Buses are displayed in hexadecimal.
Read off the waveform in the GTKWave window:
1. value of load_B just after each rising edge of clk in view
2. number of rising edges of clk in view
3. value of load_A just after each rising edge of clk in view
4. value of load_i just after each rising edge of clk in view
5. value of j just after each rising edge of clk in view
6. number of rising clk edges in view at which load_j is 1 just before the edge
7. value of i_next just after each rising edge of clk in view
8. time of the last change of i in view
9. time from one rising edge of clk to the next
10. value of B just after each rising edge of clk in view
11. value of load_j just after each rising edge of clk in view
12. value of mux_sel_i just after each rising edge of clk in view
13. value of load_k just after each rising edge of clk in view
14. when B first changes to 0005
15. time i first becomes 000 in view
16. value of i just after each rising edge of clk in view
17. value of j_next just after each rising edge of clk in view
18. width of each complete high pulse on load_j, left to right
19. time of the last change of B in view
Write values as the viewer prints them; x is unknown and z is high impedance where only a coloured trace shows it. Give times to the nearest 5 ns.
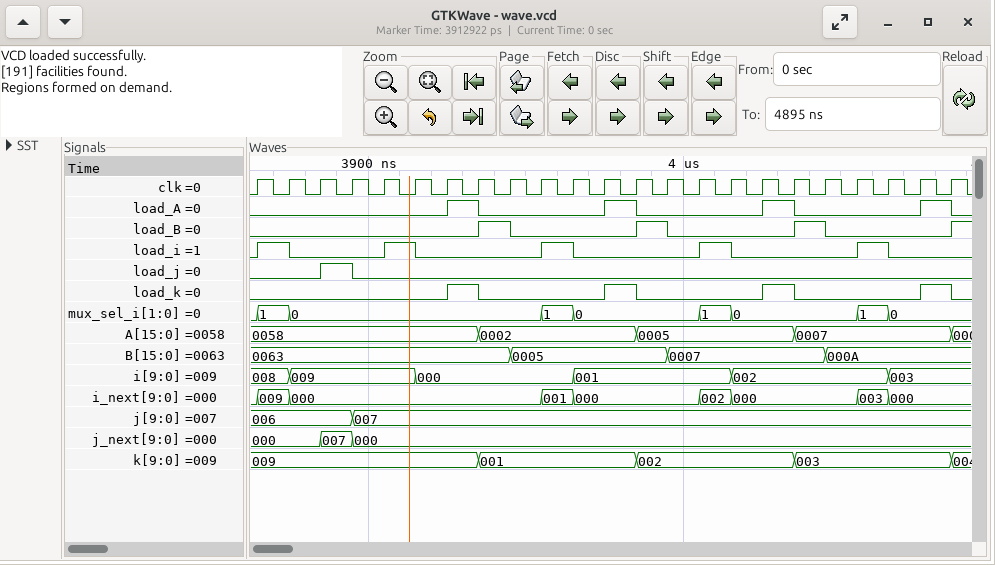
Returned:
0 0 0 0 0 0 0 1 0 0 0 0 1 0 0 0 0 1 0 0 0 0 1
23
0 0 0 0 0 0 1 0 0 0 0 1 0 0 0 0 1 0 0 0 0 1 0
1 0 0 0 1 0 0 0 0 1 0 0 0 0 1 0 0 0 0 1 0 0 0
006, 006, 006, 007, 007, 007, 007, 007, 007, 007, 007, 007, 007, 007, 007, 007, 007, 007, 007, 007, 007, 007, 007
1
009, 000, 000, 000, 000, 000, 000, 000, 000, 001, 000, 000, 000, 000, 002, 000, 000, 000, 000, 003, 000, 000, 000
4065 ns
10 ns
0063, 0063, 0063, 0063, 0063, 0063, 0063, 0063, 0005, 0005, 0005, 0005, 0005, 0007, 0007, 0007, 0007, 0007, 000A, 000A, 000A, 000A, 000A
0 0 1 0 0 0 0 0 0 0 0 0 0 0 0 0 0 0 0 0 0 0 0
1, 0, 0, 0, 0, 0, 0, 0, 0, 1, 0, 0, 0, 0, 1, 0, 0, 0, 0, 1, 0, 0, 0
0 0 0 0 0 0 1 0 0 0 0 1 0 0 0 0 1 0 0 0 0 1 0
3945 ns
3915 ns
008, 009, 009, 009, 009, 000, 000, 000, 000, 000, 001, 001, 001, 001, 001, 002, 002, 002, 002, 002, 003, 003, 003
000, 000, 007, 000, 000, 000, 000, 000, 000, 000, 000, 000, 000, 000, 000, 000, 000, 000, 000, 000, 000, 000, 000
10 ns
4045 ns
